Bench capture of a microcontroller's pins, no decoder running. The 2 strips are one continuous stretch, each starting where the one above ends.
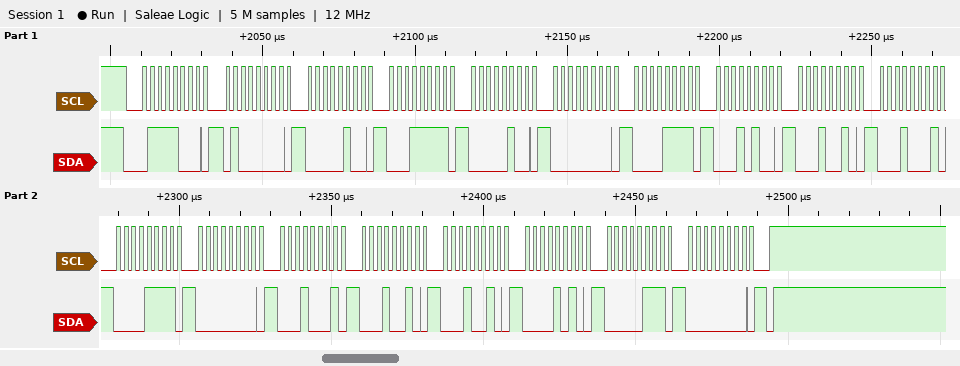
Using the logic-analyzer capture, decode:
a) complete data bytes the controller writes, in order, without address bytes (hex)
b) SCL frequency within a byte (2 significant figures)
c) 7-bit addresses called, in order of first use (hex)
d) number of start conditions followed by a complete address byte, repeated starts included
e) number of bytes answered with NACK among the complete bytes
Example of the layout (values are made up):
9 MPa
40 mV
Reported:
40 04 1F 04 00 0F 14 12 11 0F 00 11 12 12 0A 07 00
400 kHz
0x3C
1
0
